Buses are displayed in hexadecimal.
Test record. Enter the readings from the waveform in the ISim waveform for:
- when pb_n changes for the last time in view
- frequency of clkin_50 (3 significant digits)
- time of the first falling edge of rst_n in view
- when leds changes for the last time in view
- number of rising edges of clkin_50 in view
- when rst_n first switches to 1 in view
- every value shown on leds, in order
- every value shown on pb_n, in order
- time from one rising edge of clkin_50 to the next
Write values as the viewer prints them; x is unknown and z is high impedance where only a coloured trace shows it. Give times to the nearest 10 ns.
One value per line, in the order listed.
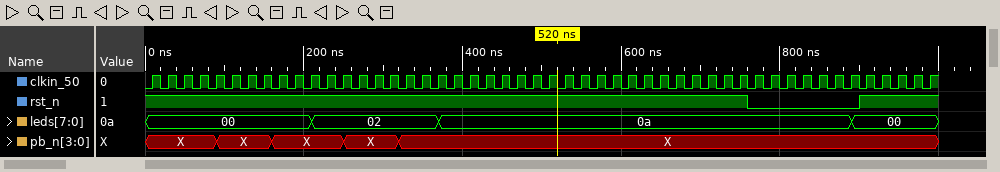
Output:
320 ns
50.0 MHz
760 ns
890 ns
50
900 ns
00, 02, 0a, 00
X, X, X, X, X
20 ns
